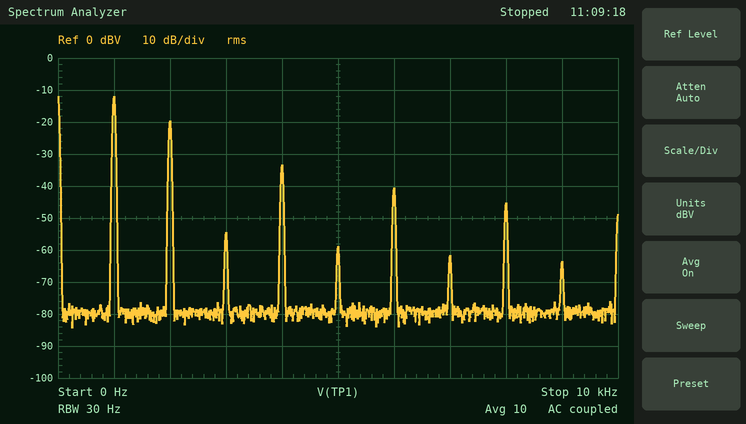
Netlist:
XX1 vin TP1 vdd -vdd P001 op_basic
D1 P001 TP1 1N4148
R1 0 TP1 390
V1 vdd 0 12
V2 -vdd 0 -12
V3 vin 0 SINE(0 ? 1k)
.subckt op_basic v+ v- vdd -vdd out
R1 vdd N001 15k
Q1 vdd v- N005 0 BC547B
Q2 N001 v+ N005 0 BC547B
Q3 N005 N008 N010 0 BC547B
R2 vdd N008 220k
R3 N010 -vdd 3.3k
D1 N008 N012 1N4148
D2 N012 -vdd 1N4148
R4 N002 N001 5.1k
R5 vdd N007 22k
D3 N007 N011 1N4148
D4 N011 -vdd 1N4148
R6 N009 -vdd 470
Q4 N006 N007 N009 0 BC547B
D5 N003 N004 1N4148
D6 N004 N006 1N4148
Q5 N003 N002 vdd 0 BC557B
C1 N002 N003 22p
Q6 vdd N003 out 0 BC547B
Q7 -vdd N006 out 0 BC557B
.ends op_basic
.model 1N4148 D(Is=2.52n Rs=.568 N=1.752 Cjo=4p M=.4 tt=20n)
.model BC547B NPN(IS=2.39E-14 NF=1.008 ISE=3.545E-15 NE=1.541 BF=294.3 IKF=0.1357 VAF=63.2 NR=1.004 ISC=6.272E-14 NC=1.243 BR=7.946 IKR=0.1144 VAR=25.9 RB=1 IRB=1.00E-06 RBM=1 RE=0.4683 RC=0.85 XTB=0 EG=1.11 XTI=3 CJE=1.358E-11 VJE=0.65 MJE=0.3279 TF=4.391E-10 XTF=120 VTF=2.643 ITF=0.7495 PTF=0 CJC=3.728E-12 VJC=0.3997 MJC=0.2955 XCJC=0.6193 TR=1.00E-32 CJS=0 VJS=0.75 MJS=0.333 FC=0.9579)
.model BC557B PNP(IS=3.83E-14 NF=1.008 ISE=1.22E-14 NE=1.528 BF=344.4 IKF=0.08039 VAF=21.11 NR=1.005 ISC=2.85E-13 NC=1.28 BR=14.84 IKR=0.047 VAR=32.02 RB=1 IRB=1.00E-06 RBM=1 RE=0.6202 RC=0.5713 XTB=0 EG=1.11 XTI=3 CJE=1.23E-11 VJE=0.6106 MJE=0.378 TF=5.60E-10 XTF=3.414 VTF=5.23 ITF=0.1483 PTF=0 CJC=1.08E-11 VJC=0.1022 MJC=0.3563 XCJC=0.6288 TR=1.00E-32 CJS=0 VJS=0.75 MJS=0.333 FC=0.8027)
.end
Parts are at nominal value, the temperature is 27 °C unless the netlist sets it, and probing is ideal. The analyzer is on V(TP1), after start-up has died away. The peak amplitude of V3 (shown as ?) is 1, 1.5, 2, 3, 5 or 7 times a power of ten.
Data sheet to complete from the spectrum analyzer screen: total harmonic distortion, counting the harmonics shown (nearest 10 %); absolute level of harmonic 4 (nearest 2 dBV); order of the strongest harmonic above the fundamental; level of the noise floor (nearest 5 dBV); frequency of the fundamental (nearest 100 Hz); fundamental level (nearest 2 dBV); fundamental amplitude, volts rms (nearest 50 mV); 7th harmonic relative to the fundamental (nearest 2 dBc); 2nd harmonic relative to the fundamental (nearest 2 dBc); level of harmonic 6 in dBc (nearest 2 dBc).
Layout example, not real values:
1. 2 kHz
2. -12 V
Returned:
1. 40 %
2. -34 dBV
3. 2
4. -80 dBV
5. 1.0 kHz
6. -12 dBV
7. 250 mV
8. -50 dBc
9. -8 dBc
10. -28 dBc
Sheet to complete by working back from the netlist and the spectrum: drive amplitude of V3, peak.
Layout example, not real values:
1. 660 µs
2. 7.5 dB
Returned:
1. 700 mV
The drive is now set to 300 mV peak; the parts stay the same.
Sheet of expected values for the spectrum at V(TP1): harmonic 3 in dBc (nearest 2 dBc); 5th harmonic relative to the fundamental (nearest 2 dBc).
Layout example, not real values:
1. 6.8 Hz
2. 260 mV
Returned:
1. -36 dBc
2. -40 dBc
